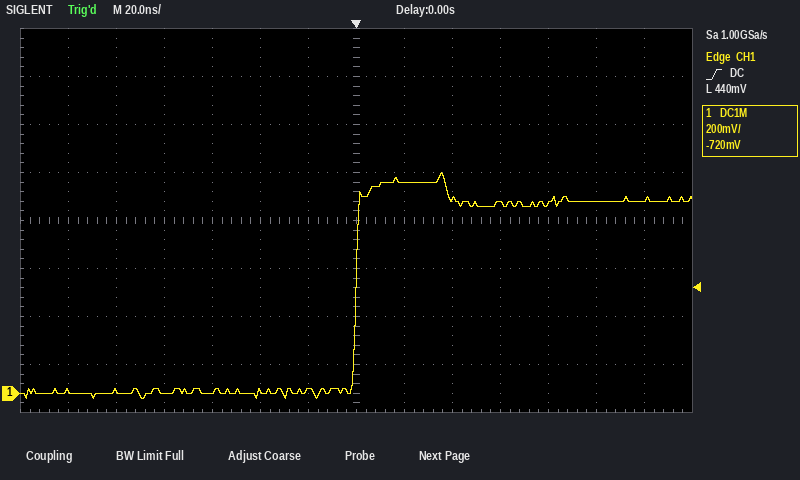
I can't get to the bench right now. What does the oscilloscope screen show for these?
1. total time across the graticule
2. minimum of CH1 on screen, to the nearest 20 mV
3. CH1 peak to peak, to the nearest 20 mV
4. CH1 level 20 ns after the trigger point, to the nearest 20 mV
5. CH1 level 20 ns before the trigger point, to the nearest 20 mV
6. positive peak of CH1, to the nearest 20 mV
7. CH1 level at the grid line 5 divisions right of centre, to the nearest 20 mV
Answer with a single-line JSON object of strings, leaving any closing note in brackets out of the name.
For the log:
{"total time across the graticule": "280 ns", "minimum of CH1 on screen, to the nearest 20 mV": "-20 mV", "CH1 peak to peak, to the nearest 20 mV": "940 mV", "CH1 level 20 ns after the trigger point, to the nearest 20 mV": "880 mV", "CH1 level 20 ns before the trigger point, to the nearest 20 mV": "20 mV", "positive peak of CH1, to the nearest 20 mV": "920 mV", "CH1 level at the grid line 5 divisions right of centre, to the nearest 20 mV": "800 mV"}
